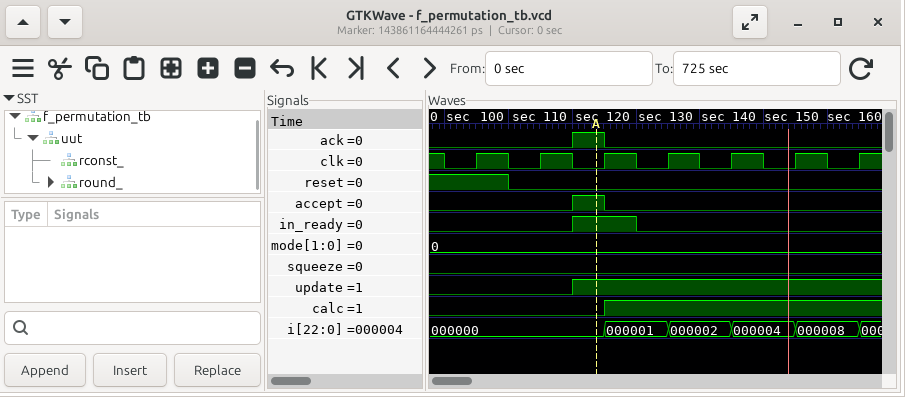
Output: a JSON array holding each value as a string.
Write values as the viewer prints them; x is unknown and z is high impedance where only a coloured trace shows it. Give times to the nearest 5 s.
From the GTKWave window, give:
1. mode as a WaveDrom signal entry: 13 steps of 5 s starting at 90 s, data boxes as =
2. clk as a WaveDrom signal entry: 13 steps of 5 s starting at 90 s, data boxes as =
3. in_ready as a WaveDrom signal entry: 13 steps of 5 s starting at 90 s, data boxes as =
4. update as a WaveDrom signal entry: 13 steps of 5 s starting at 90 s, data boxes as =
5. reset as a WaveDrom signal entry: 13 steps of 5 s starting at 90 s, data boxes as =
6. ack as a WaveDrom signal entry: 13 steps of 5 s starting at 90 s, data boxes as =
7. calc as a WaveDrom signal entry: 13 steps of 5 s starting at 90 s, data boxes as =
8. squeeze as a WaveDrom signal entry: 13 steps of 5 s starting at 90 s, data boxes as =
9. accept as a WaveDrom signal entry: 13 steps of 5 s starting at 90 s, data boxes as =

["{name: 'mode', wave: '=............', data: '0'}", "{name: 'clk', wave: '0101010101010'}", "{name: 'in_ready', wave: '0...1.0......'}", "{name: 'update', wave: '0...1........'}", "{name: 'reset', wave: '1.0..........'}", "{name: 'ack', wave: '0...10.......'}", "{name: 'calc', wave: '0....1.......'}", "{name: 'squeeze', wave: '0............'}", "{name: 'accept', wave: '0...10.......'}"]
